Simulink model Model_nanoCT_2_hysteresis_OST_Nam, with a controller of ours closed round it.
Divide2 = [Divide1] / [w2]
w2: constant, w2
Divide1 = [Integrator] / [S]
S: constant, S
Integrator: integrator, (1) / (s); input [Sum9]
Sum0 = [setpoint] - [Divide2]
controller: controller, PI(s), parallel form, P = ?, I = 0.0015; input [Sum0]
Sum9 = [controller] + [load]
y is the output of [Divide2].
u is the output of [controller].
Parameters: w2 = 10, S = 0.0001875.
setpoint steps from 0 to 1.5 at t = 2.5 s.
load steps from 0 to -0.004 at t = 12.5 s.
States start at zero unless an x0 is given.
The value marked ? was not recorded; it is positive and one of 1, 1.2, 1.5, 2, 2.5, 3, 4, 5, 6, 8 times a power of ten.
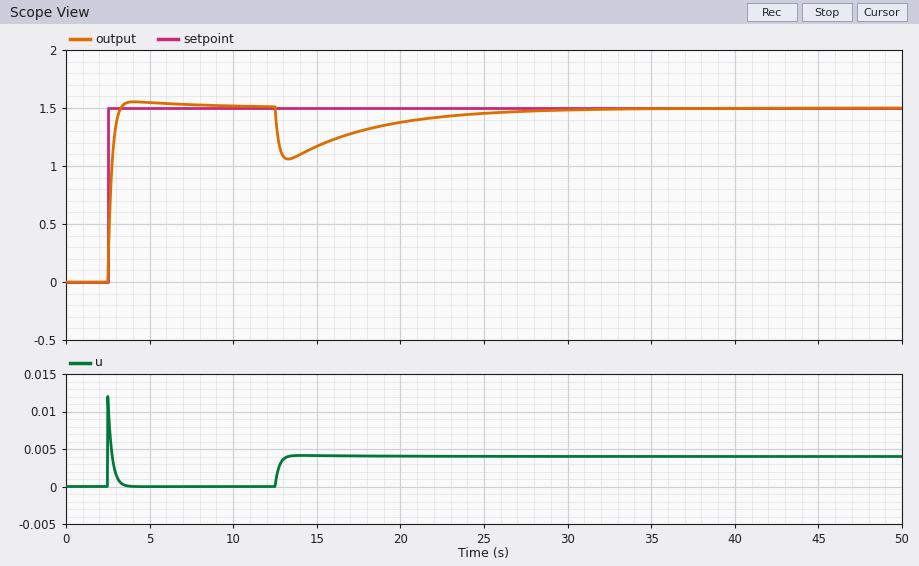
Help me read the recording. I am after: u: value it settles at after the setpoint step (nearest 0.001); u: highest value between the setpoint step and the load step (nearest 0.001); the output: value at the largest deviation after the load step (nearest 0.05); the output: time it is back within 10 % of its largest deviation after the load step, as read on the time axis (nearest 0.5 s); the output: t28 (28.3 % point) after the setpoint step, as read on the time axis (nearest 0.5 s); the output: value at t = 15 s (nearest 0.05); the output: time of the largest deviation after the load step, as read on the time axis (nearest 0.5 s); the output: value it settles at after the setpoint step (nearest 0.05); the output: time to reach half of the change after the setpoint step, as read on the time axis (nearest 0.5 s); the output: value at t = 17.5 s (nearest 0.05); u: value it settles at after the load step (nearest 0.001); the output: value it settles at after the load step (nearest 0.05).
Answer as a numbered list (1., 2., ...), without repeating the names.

1. 0.000
2. 0.012
3. 1.05
4. 25.0 s
5. 2.5 s
6. 1.15
7. 13.5 s
8. 1.50
9. 2.5 s
10. 1.30
11. 0.004
12. 1.50
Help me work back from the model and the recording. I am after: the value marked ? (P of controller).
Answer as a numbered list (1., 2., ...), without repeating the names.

1. 0.008
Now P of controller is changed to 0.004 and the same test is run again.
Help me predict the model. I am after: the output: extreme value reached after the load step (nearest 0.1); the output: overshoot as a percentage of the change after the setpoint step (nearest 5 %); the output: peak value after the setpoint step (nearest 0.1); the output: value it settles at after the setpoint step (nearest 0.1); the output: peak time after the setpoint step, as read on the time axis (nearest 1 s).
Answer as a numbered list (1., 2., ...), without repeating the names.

1. 0.7
2. 10 %
3. 1.7
4. 1.5
5. 5 s
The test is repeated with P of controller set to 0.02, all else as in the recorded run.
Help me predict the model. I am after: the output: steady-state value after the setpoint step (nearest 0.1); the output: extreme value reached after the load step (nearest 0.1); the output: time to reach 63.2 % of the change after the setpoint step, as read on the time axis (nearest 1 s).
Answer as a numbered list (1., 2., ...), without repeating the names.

1. 1.5
2. 1.3
3. 3 s
